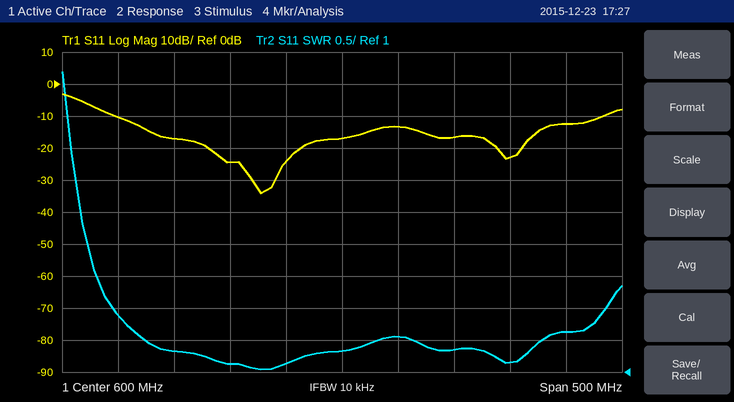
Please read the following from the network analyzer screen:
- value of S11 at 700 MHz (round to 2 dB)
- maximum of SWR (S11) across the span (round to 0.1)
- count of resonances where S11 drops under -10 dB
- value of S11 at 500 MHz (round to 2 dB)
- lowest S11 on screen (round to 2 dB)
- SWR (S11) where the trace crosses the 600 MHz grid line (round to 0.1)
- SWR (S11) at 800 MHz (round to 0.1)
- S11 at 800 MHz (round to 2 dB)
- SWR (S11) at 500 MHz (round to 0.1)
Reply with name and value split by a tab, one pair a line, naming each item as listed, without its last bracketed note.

value of S11 at 700 MHz	-16 dB
maximum of SWR (S11) across the span	5.7
count of resonances where S11 drops under -10 dB	2
value of S11 at 500 MHz	-24 dB
lowest S11 on screen	-34 dB
SWR (S11) where the trace crosses the 600 MHz grid line	1.3
SWR (S11) at 800 MHz	1.6
S11 at 800 MHz	-12 dB
SWR (S11) at 500 MHz	1.1
